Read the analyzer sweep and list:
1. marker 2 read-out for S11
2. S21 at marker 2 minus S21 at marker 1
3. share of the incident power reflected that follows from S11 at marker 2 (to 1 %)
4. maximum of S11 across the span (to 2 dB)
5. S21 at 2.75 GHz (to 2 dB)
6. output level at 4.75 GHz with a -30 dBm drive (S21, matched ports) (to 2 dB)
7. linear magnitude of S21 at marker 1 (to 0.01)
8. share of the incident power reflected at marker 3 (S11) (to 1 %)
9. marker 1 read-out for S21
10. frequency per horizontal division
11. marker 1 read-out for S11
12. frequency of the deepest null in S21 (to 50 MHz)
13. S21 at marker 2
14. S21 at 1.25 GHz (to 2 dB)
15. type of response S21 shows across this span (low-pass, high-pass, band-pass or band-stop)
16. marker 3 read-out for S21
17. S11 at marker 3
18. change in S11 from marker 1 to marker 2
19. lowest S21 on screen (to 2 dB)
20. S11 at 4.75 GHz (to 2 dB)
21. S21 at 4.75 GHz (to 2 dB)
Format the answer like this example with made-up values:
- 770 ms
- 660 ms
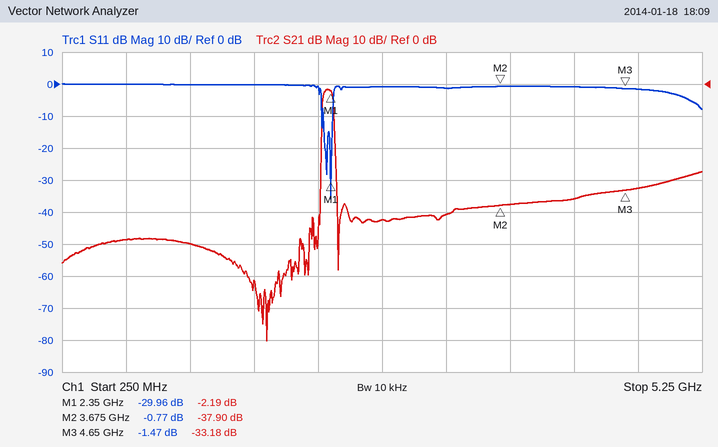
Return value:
- -0.77 dB
- -35.71 dB
- 84 %
- 0 dB
- -42 dB
- -62 dBm
- 0.78
- 71 %
- -2.19 dB
- 500 MHz
- -29.96 dB
- 1.85 GHz
- -37.90 dB
- -50 dB
- band-pass
- -33.18 dB
- -1.47 dB
- 29.19 dB
- -80 dB
- -2 dB
- -32 dB
